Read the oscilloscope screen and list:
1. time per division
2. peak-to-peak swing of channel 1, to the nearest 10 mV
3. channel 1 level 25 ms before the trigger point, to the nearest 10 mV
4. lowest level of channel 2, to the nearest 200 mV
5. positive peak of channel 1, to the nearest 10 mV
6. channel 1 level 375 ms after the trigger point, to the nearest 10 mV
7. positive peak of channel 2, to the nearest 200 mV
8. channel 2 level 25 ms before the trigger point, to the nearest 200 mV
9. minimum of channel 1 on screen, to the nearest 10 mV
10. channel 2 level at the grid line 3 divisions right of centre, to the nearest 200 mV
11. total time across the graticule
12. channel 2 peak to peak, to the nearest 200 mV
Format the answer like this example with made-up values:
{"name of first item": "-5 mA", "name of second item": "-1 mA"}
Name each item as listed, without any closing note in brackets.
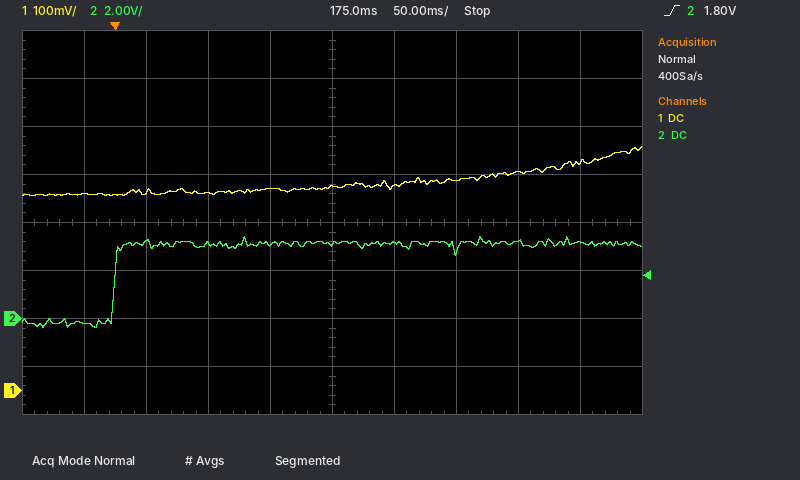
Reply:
{"time per division": "50 ms", "peak-to-peak swing of channel 1, to the nearest 10 mV": "100 mV", "channel 1 level 25 ms before the trigger point, to the nearest 10 mV": "410 mV", "lowest level of channel 2, to the nearest 200 mV": "-400 mV", "positive peak of channel 1, to the nearest 10 mV": "510 mV", "channel 1 level 375 ms after the trigger point, to the nearest 10 mV": "480 mV", "positive peak of channel 2, to the nearest 200 mV": "3.4 V", "channel 2 level 25 ms before the trigger point, to the nearest 200 mV": "-200 mV", "minimum of channel 1 on screen, to the nearest 10 mV": "410 mV", "channel 2 level at the grid line 3 divisions right of centre, to the nearest 200 mV": "3.2 V", "total time across the graticule": "500 ms", "channel 2 peak to peak, to the nearest 200 mV": "3.8 V"}
